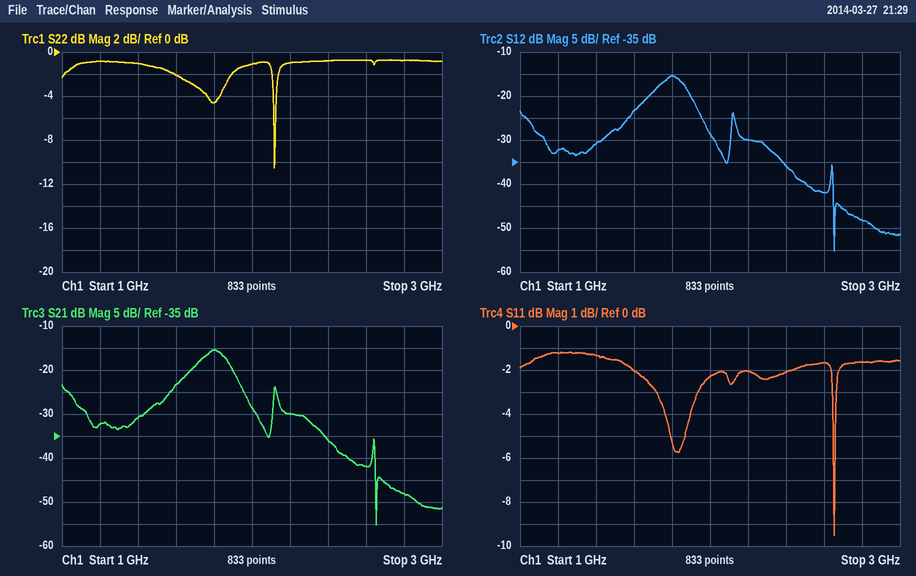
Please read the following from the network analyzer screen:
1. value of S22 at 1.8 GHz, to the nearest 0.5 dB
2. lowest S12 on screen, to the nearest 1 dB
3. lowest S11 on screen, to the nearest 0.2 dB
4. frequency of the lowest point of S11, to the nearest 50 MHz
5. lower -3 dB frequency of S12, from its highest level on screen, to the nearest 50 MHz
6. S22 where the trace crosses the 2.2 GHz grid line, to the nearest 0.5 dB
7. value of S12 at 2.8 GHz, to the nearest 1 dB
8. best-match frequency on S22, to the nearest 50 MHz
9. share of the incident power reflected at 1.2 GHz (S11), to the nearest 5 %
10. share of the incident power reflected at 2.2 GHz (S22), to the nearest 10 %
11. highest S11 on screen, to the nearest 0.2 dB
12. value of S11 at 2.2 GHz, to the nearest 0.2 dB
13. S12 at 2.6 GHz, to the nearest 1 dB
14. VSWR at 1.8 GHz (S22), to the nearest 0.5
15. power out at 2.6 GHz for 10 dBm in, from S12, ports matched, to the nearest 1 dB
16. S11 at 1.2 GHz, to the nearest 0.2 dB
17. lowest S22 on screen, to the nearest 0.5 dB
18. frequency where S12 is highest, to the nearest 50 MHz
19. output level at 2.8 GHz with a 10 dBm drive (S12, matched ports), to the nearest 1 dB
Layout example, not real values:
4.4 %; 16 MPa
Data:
-4.5 dB; -55 dB; -9.6 dB; 2.65 GHz; 1.70 GHz; -1.0 dB; -48 dB; 2.10 GHz; 75 %; 80 %; -1.2 dB; -2.0 dB; -42 dB; 4.0; -32 dBm; -1.2 dB; -10.5 dB; 1.80 GHz; -38 dBm
